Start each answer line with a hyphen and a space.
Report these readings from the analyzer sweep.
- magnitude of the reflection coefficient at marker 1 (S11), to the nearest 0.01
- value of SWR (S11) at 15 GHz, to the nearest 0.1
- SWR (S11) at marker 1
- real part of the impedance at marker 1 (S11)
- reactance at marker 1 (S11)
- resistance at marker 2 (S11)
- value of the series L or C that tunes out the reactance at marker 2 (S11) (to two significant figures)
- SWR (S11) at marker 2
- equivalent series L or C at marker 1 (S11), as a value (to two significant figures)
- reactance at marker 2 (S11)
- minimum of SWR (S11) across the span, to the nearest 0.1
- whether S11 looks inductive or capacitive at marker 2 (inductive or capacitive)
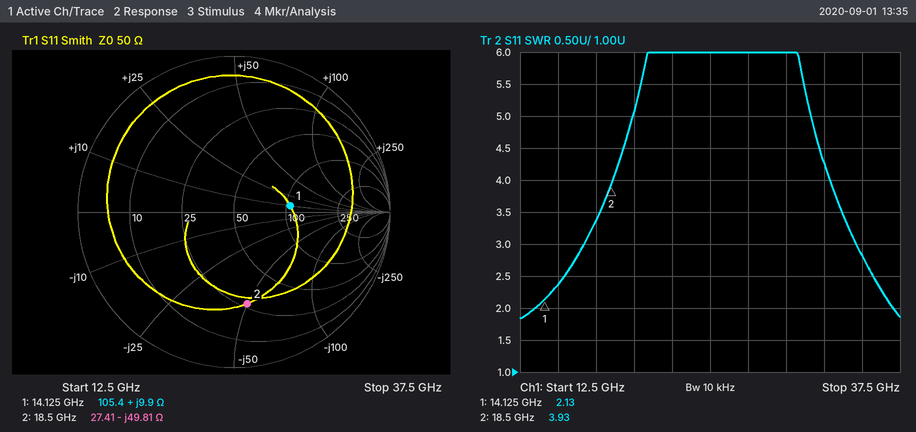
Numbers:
- 0.36
- 2.4
- 2.13
- 105.4 Ω
- +9.9 Ω
- 27.41 Ω
- 430 pH
- 3.93
- 110 pH
- -49.81 Ω
- 1.8
- capacitive
